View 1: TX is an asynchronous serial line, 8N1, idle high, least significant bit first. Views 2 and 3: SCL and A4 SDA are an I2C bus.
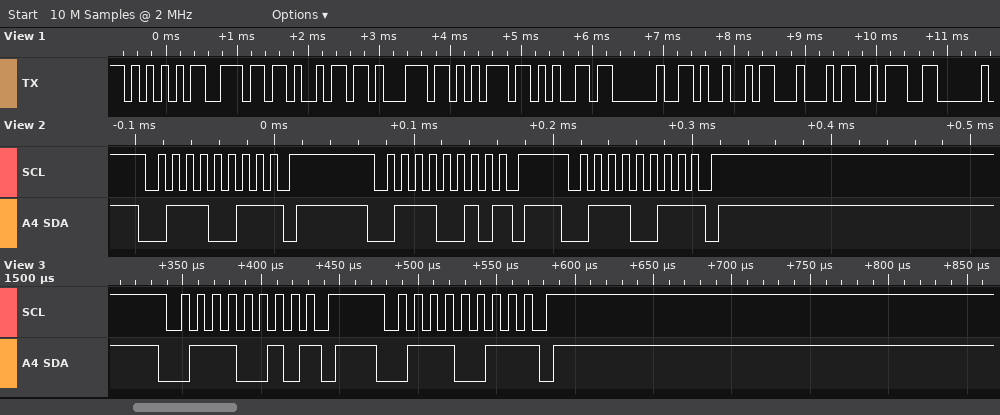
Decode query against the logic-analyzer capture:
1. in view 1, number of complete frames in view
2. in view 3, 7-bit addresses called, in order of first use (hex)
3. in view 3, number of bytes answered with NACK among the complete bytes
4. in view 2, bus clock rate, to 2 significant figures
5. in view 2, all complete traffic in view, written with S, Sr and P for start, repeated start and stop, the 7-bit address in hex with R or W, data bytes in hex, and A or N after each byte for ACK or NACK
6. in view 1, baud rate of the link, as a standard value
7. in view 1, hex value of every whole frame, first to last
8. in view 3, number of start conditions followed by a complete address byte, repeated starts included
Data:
10
0x39
2
100 kHz
S 39R N P S 39W N P S 39R N P
9600 baud
0x55 0x6E 0x69 0x71 0x75 0x65 0x20 0x49 0x44 0x3A
2
